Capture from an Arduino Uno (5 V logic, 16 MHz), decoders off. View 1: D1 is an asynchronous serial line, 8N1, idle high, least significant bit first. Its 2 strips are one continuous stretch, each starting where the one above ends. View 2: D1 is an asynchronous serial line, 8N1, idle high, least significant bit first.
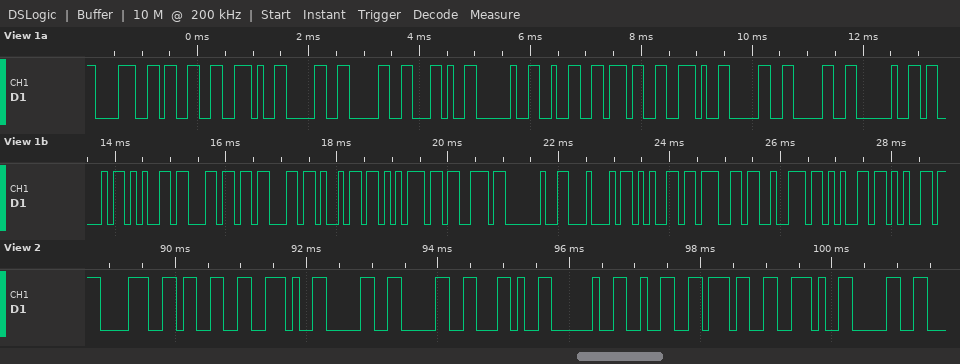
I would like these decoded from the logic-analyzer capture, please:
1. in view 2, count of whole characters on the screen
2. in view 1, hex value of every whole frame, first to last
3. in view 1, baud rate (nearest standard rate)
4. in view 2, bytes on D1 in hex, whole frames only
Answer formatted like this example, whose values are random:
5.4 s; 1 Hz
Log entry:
11; 38 33 2E 30 30 2C 20 32 37 2E 30 30 20 43 65 6C 63 69 75 73 20 44 65 67 72 65 65; 9600 baud; 38 33 2E 30 30 2C 20 32 37 2E 30
